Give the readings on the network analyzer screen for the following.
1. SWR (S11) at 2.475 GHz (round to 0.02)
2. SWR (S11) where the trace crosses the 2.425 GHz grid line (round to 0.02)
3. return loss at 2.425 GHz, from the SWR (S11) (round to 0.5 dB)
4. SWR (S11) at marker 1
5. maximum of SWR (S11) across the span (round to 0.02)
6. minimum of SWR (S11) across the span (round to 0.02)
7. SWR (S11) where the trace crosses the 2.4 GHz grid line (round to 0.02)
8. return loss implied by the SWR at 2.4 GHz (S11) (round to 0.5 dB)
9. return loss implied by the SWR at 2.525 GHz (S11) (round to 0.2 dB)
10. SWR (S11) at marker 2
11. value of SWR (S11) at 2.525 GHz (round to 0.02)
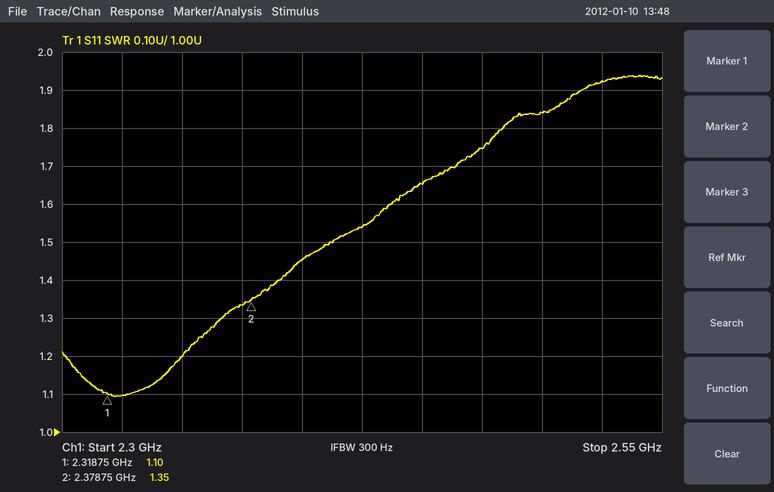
1.74
1.54
13.5 dB
1.10
1.94
1.10
1.46
14.5 dB
10.0 dB
1.35
1.92
